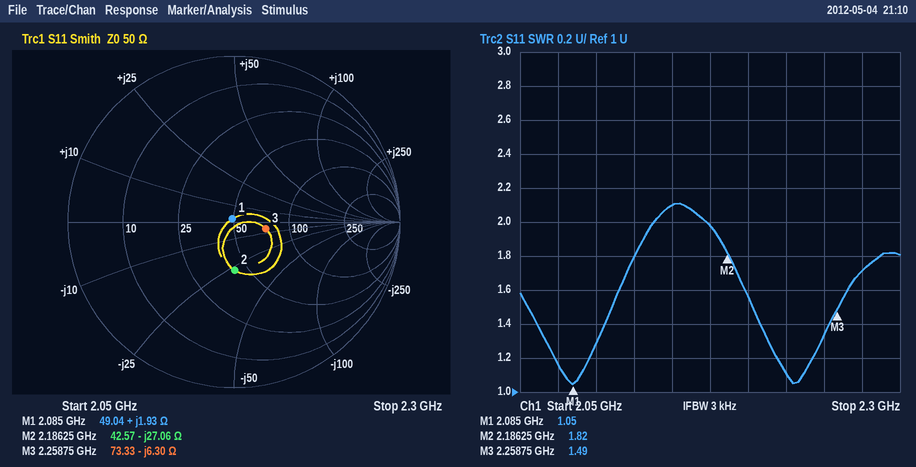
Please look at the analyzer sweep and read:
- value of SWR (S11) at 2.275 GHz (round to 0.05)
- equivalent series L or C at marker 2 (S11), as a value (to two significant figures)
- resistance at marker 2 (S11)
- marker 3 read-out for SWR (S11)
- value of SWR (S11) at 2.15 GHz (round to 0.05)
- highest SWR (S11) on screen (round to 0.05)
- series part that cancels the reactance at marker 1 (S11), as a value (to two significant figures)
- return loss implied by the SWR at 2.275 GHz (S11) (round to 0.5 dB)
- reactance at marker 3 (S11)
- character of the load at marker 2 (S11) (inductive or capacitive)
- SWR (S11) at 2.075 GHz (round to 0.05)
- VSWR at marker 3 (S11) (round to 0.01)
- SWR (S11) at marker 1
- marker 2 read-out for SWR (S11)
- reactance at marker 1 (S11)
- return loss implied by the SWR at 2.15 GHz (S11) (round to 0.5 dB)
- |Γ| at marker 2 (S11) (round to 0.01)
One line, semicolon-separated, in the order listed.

1.70; 2.7 pF; 42.57 Ω; 1.49; 2.10; 2.10; 40 pF; 11.5 dB; -6.30 Ω; capacitive; 1.15; 1.49; 1.05; 1.82; +1.93 Ω; 9.0 dB; 0.29
